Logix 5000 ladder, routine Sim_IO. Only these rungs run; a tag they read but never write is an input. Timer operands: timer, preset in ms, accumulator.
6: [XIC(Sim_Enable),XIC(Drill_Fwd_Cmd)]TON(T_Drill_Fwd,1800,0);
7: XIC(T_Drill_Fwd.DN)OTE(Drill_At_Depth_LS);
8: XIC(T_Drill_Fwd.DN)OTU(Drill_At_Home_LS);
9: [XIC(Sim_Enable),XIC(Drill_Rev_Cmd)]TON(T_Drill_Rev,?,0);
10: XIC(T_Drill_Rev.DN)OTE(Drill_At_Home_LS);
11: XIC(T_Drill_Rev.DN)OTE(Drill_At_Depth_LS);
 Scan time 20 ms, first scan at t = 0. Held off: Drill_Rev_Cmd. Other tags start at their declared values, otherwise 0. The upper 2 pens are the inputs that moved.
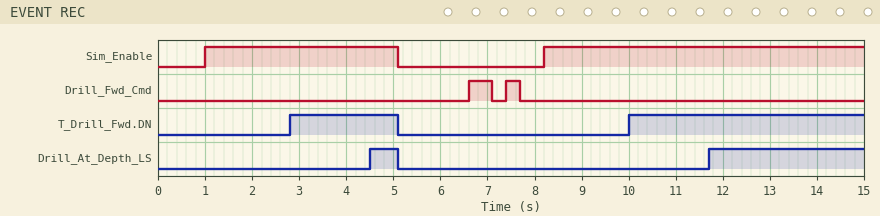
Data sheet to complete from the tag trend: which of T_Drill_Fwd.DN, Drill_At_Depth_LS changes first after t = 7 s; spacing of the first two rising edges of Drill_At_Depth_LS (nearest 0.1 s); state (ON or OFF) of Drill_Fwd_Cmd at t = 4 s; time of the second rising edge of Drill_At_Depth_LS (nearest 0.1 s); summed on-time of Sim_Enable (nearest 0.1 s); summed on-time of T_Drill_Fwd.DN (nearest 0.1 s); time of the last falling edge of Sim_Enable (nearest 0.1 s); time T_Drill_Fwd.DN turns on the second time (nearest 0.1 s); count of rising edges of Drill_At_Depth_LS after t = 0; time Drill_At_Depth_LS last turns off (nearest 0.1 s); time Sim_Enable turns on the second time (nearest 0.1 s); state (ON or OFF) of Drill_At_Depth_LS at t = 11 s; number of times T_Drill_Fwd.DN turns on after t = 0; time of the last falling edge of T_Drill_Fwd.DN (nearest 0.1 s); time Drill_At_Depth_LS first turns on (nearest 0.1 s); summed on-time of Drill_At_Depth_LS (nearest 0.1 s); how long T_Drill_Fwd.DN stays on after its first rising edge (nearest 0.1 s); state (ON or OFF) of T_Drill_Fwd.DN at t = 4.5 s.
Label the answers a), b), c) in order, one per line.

a) T_Drill_Fwd.DN
b) 7.2 s
c) OFF
d) 11.7 s
e) 10.9 s
f) 7.3 s
g) 5.1 s
h) 10.0 s
i) 2
j) 5.1 s
k) 8.2 s
l) OFF
m) 2
n) 5.1 s
o) 4.5 s
p) 3.9 s
q) 2.3 s
r) ON
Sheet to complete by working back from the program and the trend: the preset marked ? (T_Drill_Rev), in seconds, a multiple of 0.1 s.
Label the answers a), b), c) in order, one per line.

a) 3.5 s
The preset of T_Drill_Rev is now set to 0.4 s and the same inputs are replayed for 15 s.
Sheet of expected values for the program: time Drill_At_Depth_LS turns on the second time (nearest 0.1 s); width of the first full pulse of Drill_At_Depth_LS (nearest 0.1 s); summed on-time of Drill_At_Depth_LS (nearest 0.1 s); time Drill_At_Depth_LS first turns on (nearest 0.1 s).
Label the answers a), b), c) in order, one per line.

a) 8.6 s
b) 3.7 s
c) 10.1 s
d) 1.4 s
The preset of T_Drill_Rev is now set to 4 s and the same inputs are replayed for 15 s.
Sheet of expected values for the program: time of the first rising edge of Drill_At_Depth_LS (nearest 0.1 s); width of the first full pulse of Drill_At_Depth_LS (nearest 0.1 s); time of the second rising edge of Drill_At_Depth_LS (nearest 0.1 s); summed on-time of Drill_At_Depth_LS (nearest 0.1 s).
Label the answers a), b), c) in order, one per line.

a) 5.0 s
b) 0.1 s
c) 12.2 s
d) 2.9 s
